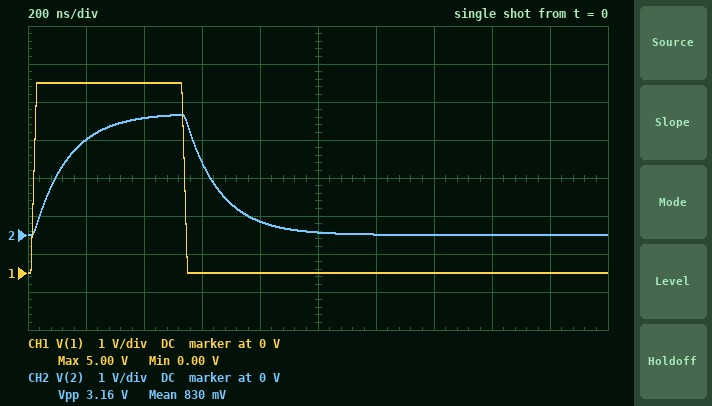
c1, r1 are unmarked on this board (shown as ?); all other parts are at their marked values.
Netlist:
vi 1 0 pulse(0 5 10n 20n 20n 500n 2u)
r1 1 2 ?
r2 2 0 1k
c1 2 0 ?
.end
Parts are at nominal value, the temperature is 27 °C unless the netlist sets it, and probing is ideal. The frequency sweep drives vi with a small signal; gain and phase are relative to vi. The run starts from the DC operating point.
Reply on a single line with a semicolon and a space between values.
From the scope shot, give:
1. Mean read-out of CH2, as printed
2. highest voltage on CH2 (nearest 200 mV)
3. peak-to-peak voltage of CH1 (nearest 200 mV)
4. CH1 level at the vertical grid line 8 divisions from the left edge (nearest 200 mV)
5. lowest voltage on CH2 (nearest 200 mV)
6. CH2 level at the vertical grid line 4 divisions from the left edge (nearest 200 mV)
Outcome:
830 mV; 3.2 V; 5.0 V; 0 V; 0 V; 400 mV
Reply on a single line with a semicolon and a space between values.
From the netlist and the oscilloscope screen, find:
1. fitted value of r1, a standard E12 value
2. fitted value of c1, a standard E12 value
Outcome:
560 Ω; 330 pF
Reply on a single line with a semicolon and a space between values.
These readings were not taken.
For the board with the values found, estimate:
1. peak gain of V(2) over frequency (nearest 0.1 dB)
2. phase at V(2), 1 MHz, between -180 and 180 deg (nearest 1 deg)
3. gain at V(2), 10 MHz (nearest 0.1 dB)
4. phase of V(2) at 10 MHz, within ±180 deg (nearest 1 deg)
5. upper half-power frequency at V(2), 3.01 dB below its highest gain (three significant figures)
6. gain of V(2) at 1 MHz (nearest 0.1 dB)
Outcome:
-3.9 dB; -37 deg; -21.4 dB; -82 deg; 1.34 MHz; -5.8 dB
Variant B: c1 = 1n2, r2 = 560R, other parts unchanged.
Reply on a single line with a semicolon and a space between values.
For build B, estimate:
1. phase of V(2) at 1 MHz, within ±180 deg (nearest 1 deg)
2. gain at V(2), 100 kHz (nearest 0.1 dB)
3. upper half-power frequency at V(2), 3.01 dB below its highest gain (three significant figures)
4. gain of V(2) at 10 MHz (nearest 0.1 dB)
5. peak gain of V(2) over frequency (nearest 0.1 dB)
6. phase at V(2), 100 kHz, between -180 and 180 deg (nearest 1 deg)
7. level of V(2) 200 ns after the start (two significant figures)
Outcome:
-65 deg; -6.2 dB; 474 kHz; -32.5 dB; -6.0 dB; -12 deg; 1.0 V
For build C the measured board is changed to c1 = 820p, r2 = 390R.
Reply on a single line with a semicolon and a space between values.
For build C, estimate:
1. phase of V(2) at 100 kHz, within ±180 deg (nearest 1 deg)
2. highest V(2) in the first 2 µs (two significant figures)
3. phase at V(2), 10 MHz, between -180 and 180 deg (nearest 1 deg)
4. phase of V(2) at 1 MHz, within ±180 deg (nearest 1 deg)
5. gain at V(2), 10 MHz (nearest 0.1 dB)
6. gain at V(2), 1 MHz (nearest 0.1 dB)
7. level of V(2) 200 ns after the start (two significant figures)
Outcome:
-7 deg; 1.9 V; -85 deg; -50 deg; -29.2 dB; -11.5 dB; 1.3 V
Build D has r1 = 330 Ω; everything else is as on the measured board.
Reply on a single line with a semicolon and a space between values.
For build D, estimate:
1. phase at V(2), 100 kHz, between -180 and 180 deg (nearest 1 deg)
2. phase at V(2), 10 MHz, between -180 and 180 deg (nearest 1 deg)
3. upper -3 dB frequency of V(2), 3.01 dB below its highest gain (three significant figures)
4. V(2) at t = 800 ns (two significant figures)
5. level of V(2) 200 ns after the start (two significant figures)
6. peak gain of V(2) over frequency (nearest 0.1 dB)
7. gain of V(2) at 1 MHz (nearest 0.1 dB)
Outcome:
-3 deg; -79 deg; 1.94 MHz; 160 mV; 3.3 V; -2.5 dB; -3.5 dB
